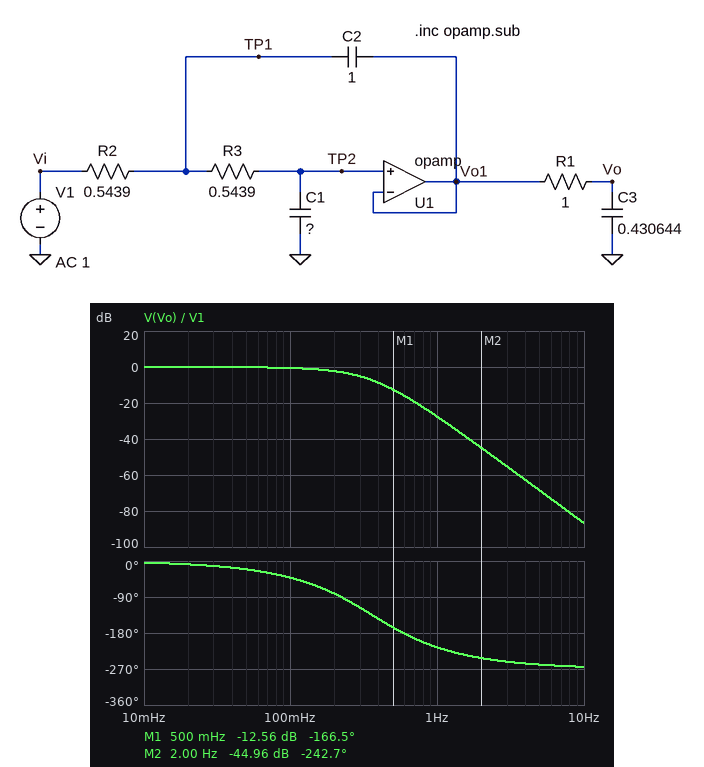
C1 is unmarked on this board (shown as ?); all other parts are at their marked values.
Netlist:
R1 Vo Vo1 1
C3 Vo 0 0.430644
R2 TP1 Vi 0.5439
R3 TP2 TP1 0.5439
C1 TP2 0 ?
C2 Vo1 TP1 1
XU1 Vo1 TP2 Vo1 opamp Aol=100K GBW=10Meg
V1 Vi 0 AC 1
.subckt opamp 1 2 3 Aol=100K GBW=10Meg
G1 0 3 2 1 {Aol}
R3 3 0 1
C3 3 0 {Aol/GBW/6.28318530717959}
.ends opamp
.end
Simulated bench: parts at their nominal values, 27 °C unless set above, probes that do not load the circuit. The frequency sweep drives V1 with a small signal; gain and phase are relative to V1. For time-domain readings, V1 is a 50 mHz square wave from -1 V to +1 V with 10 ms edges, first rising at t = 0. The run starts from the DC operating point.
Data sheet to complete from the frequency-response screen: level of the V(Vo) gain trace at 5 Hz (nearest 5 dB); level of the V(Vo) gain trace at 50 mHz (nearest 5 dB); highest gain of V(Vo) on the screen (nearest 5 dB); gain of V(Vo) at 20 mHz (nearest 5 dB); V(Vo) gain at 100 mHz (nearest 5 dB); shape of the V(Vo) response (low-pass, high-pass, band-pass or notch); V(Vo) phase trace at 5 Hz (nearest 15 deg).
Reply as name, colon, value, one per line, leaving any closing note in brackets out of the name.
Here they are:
level of the V(Vo) gain trace at 5 Hz: -70 dB
level of the V(Vo) gain trace at 50 mHz: 0 dB
highest gain of V(Vo) on the screen: 0 dB
gain of V(Vo) at 20 mHz: 0 dB
V(Vo) gain at 100 mHz: 0 dB
shape of the V(Vo) response: low-pass
V(Vo) phase trace at 5 Hz: -255 deg
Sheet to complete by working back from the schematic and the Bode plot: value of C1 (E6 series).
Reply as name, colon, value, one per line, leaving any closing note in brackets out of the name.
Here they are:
value of C1: 680 mF
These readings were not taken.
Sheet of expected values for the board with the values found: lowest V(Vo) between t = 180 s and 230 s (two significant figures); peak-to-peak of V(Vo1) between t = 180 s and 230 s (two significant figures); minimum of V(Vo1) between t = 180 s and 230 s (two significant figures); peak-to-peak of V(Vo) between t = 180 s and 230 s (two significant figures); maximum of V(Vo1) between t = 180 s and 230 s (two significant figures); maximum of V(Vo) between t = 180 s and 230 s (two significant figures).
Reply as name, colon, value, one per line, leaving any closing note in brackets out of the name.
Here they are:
lowest V(Vo) between t = 180 s and 230 s: -1.0 V
peak-to-peak of V(Vo1) between t = 180 s and 230 s: 2.0 V
minimum of V(Vo1) between t = 180 s and 230 s: -1.0 V
peak-to-peak of V(Vo) between t = 180 s and 230 s: 2.0 V
maximum of V(Vo1) between t = 180 s and 230 s: 1.0 V
maximum of V(Vo) between t = 180 s and 230 s: 1.0 V
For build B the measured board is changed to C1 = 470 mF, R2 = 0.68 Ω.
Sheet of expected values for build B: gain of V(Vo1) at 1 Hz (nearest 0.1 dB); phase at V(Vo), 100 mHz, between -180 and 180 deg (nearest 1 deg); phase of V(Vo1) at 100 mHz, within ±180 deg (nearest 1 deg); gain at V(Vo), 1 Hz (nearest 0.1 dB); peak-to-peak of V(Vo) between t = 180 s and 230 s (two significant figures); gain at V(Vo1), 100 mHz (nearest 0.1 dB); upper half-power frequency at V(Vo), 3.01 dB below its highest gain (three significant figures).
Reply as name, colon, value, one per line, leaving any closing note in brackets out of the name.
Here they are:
gain of V(Vo1) at 1 Hz: -16.8 dB
phase at V(Vo), 100 mHz, between -180 and 180 deg: -36 deg
phase of V(Vo1) at 100 mHz, within ±180 deg: -21 deg
gain at V(Vo), 1 Hz: -26.0 dB
peak-to-peak of V(Vo) between t = 180 s and 230 s: 2.1 V
gain at V(Vo1), 100 mHz: 0 dB
upper half-power frequency at V(Vo), 3.01 dB below its highest gain: 285 mHz
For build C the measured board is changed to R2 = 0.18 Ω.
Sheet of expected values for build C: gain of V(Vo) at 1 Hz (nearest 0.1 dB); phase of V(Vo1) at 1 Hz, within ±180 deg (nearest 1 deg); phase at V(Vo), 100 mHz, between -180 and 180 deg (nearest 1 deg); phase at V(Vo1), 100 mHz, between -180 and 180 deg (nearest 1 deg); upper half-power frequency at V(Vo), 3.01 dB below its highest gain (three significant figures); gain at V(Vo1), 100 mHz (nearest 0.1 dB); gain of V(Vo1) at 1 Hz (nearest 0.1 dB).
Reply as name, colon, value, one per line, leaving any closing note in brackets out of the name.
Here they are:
gain of V(Vo) at 1 Hz: -20.1 dB
phase of V(Vo1) at 1 Hz, within ±180 deg: -118 deg
phase at V(Vo), 100 mHz, between -180 and 180 deg: -33 deg
phase at V(Vo1), 100 mHz, between -180 and 180 deg: -18 deg
upper half-power frequency at V(Vo), 3.01 dB below its highest gain: 262 mHz
gain at V(Vo1), 100 mHz: -0.2 dB
gain of V(Vo1) at 1 Hz: -10.9 dB
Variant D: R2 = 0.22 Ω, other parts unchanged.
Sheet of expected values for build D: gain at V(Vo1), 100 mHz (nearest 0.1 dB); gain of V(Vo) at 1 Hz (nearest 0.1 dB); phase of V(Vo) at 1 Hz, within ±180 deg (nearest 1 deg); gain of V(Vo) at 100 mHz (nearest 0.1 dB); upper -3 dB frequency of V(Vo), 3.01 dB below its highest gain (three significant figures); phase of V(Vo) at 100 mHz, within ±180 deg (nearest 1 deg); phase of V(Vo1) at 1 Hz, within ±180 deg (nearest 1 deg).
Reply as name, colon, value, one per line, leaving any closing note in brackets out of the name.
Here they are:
gain at V(Vo1), 100 mHz: -0.2 dB
gain of V(Vo) at 1 Hz: -21.1 dB
phase of V(Vo) at 1 Hz, within ±180 deg: 166 deg
gain of V(Vo) at 100 mHz: -0.5 dB
upper -3 dB frequency of V(Vo), 3.01 dB below its highest gain: 261 mHz
phase of V(Vo) at 100 mHz, within ±180 deg: -34 deg
phase of V(Vo1) at 1 Hz, within ±180 deg: -124 deg
